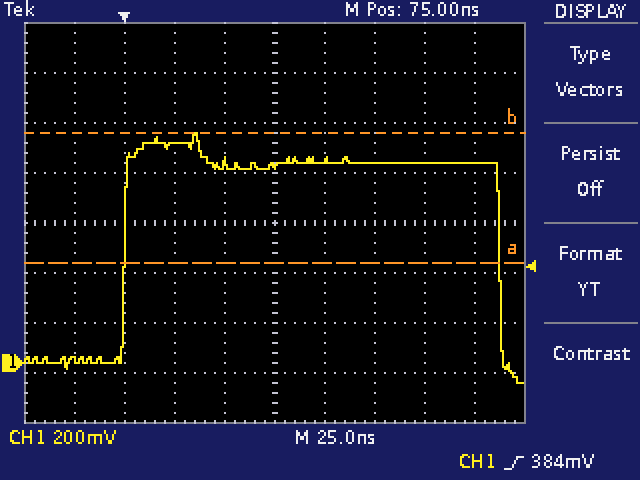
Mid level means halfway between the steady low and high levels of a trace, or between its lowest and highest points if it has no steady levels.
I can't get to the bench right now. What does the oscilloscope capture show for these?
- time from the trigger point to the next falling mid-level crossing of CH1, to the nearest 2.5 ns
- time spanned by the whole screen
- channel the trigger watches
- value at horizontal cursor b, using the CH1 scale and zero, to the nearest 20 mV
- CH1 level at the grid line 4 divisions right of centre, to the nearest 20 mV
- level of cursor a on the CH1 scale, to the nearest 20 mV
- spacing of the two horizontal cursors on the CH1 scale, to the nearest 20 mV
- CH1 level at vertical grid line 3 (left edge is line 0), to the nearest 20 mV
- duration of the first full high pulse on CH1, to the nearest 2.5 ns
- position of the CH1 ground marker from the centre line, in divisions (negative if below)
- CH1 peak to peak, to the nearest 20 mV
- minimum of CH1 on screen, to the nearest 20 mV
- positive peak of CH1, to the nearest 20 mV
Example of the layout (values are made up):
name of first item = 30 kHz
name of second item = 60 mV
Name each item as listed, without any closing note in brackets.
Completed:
time from the trigger point to the next falling mid-level crossing of CH1, to the nearest 2.5 ns = 187.5 ns
time spanned by the whole screen = 250 ns
channel the trigger watches = CH1
value at horizontal cursor b, using the CH1 scale and zero, to the nearest 20 mV = 920 mV
CH1 level at the grid line 4 divisions right of centre, to the nearest 20 mV = 800 mV
level of cursor a on the CH1 scale, to the nearest 20 mV = 400 mV
spacing of the two horizontal cursors on the CH1 scale, to the nearest 20 mV = 520 mV
CH1 level at vertical grid line 3 (left edge is line 0), to the nearest 20 mV = 880 mV
duration of the first full high pulse on CH1, to the nearest 2.5 ns = 187.5 ns
position of the CH1 ground marker from the centre line, in divisions = -2.8 div
CH1 peak to peak, to the nearest 20 mV = 1.00 V
minimum of CH1 on screen, to the nearest 20 mV = -80 mV
positive peak of CH1, to the nearest 20 mV = 920 mV
